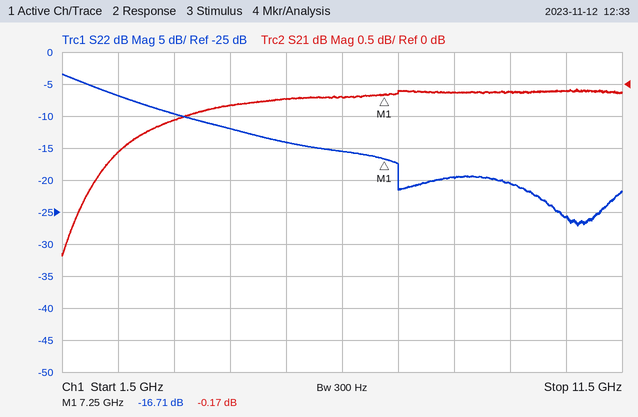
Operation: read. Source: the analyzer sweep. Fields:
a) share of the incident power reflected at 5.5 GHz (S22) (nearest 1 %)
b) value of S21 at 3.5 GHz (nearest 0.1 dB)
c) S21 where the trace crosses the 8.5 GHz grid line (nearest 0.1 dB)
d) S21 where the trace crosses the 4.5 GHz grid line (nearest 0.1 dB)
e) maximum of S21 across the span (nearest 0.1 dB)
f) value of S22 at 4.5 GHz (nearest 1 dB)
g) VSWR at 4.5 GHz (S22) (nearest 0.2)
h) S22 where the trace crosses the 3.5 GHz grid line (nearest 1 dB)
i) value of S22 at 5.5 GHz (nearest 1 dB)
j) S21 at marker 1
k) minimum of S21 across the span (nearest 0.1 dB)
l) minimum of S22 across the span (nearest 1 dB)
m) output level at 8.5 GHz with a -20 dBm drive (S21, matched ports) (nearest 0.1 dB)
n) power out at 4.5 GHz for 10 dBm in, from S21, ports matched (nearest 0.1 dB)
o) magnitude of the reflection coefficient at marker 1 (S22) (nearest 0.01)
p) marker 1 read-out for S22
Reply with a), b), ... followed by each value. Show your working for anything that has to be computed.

a) 10^(-14/10) ≈ 4 %
b) -0.6 dB
c) -0.1 dB
d) -0.3 dB
e) -0.1 dB
f) -12 dB
g) |Γ| = 10^(-12/20) = 0.2512; VSWR = (1 + 0.2512)/(1 − 0.2512) ≈ 1.67, so 1.6 to the nearest 0.2
h) -10 dB
i) -14 dB
j) -0.17 dB
k) -2.7 dB
l) -27 dB
m) -20 dBm + (-0.1 dB) = -20.1 dBm
n) 10 dBm + (-0.3 dB) = 9.7 dBm
o) 10^(-16.71/20) ≈ 0.15
p) -16.71 dB
